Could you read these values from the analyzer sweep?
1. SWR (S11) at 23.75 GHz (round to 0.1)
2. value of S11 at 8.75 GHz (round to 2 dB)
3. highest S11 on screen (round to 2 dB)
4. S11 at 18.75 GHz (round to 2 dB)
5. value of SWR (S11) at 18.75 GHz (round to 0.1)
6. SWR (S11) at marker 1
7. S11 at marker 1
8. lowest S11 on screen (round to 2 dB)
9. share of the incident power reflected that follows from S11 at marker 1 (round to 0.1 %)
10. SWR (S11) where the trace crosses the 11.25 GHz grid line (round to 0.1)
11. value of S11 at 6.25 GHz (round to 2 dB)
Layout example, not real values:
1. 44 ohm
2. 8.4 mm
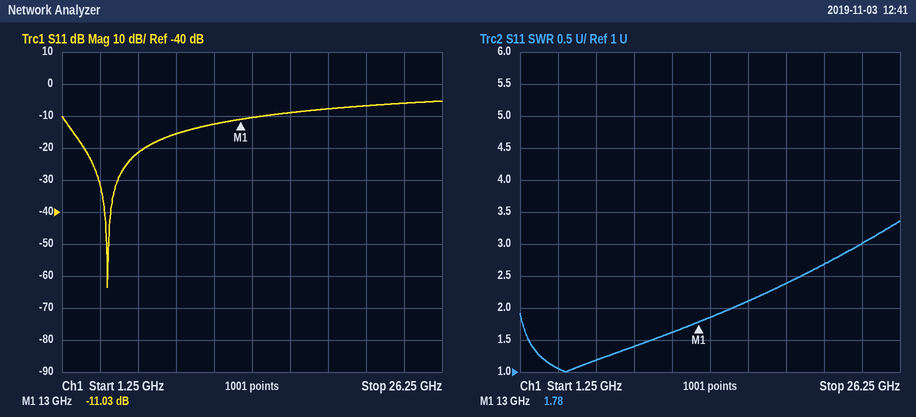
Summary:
1. 3.0
2. -16 dB
3. -6 dB
4. -8 dB
5. 2.4
6. 1.78
7. -11.03 dB
8. -64 dB
9. 7.9 %
10. 1.6
11. -22 dB
